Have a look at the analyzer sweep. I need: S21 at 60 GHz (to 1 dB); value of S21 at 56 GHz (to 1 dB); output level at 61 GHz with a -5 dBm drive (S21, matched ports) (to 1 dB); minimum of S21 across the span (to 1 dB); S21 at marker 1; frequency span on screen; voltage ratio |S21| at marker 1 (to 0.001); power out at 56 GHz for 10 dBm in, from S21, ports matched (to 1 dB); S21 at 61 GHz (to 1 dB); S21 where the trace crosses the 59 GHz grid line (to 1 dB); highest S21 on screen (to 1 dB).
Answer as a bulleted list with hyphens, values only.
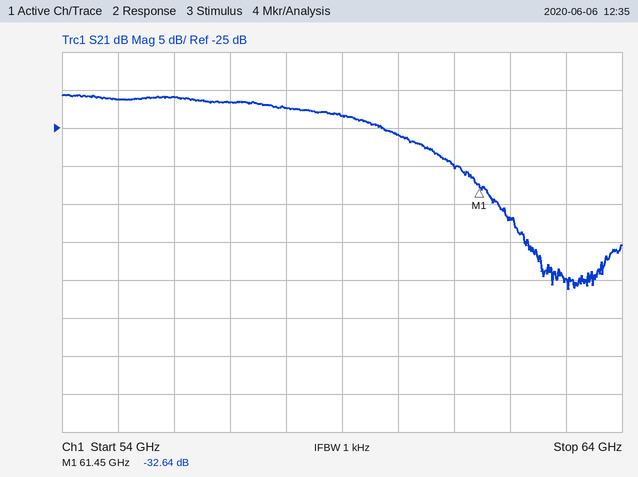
- -26 dB
- -21 dB
- -35 dBm
- -46 dB
- -32.64 dB
- 10 GHz
- 0.023
- -11 dBm
- -30 dB
- -23 dB
- -21 dB
